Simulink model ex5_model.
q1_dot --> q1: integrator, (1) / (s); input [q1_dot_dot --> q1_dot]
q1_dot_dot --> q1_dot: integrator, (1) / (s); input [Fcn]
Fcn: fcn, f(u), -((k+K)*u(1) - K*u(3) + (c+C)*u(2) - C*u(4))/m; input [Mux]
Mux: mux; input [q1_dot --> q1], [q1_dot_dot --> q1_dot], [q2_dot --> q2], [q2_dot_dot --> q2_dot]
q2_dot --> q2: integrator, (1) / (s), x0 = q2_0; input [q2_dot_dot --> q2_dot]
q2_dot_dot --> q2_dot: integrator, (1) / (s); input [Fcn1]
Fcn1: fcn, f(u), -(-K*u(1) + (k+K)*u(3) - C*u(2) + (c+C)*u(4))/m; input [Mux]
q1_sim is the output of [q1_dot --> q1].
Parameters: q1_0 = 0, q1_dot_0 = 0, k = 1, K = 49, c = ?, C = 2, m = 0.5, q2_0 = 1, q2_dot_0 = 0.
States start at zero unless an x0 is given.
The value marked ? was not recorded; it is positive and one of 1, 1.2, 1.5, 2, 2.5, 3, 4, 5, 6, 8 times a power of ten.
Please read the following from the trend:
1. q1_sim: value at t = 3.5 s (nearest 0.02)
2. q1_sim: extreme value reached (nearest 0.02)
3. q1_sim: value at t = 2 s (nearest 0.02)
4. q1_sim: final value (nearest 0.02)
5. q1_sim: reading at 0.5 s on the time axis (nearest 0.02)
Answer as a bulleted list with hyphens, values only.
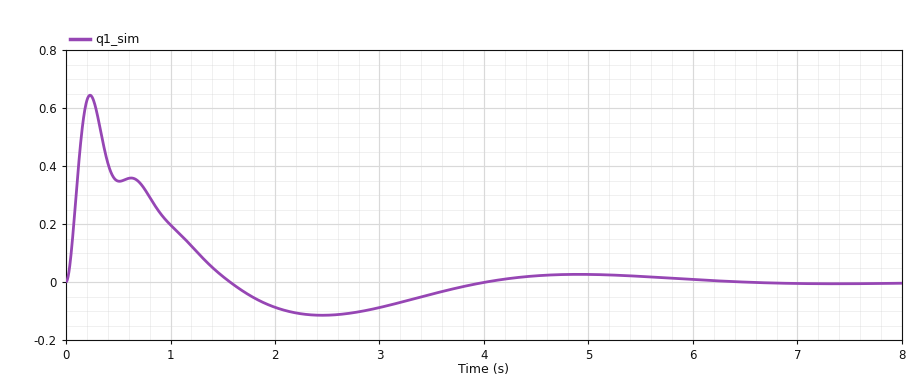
- -0.04
- 0.64
- -0.08
- 0.00
- 0.34
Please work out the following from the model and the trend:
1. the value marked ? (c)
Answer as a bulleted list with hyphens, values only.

- 0.6
